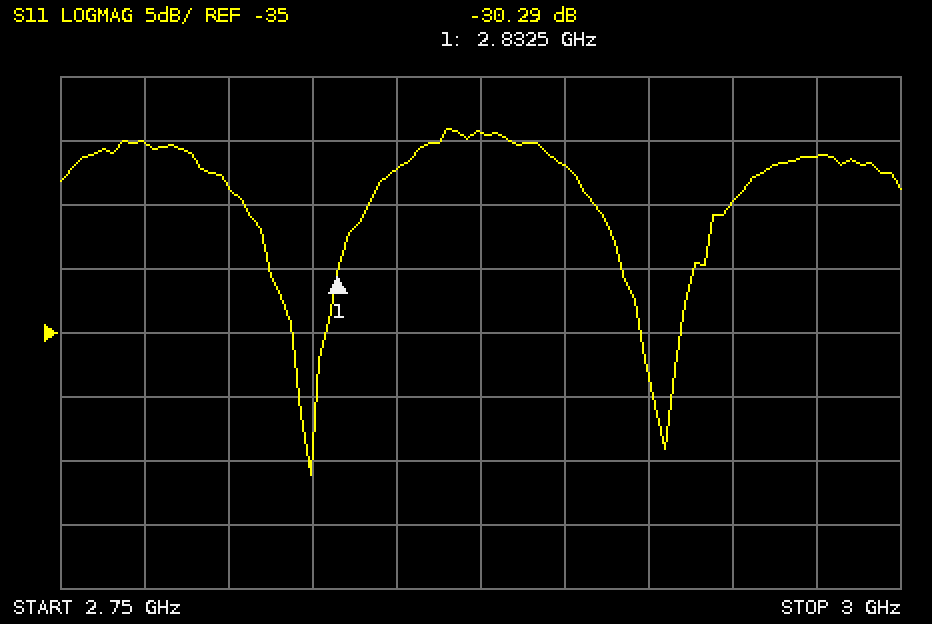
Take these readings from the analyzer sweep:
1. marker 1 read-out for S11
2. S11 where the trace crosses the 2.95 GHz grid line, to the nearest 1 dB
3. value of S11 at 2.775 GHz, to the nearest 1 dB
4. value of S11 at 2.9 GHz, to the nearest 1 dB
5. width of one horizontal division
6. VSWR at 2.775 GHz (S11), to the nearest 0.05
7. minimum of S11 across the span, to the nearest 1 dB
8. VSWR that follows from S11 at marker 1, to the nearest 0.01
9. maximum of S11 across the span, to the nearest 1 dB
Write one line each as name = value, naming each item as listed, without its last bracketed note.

marker 1 read-out for S11 = -30.29 dB
S11 where the trace crosses the 2.95 GHz grid line, to the nearest 1 dB = -25 dB
value of S11 at 2.775 GHz, to the nearest 1 dB = -20 dB
value of S11 at 2.9 GHz, to the nearest 1 dB = -22 dB
width of one horizontal division = 25 MHz
VSWR at 2.775 GHz (S11), to the nearest 0.05 = 1.20
minimum of S11 across the span, to the nearest 1 dB = -46 dB
VSWR that follows from S11 at marker 1, to the nearest 0.01 = 1.06
maximum of S11 across the span, to the nearest 1 dB = -19 dB
